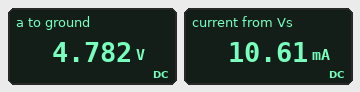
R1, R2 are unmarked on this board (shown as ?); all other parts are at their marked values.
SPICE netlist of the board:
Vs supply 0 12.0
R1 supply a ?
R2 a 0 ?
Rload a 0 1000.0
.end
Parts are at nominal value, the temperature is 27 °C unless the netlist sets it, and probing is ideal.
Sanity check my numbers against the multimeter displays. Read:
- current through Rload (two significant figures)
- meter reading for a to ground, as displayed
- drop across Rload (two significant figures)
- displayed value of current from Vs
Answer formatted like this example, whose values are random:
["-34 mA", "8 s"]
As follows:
["4.8 mA", "4.782 V", "4.8 V", "10.61 mA"]
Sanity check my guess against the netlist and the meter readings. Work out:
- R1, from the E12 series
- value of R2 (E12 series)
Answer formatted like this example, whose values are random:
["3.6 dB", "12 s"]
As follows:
["680 Ω", "820 Ω"]
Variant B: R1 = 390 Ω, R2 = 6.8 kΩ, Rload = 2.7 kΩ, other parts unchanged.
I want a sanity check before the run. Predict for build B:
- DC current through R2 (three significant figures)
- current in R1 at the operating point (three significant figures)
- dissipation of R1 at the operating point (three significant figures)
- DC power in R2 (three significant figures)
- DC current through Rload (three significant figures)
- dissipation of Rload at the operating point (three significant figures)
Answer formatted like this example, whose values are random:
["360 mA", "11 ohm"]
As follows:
["1.47 mA", "5.17 mA", "10.4 mW", "14.7 mW", "3.70 mA", "36.9 mW"]
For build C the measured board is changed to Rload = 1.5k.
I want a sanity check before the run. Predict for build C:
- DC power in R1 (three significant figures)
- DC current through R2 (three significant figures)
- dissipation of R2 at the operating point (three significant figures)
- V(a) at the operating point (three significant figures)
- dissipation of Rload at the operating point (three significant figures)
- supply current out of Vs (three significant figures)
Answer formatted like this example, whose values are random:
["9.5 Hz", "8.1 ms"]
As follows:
["66.9 mW", "6.41 mA", "33.7 mW", "5.26 V", "18.4 mW", "9.92 mA"]
